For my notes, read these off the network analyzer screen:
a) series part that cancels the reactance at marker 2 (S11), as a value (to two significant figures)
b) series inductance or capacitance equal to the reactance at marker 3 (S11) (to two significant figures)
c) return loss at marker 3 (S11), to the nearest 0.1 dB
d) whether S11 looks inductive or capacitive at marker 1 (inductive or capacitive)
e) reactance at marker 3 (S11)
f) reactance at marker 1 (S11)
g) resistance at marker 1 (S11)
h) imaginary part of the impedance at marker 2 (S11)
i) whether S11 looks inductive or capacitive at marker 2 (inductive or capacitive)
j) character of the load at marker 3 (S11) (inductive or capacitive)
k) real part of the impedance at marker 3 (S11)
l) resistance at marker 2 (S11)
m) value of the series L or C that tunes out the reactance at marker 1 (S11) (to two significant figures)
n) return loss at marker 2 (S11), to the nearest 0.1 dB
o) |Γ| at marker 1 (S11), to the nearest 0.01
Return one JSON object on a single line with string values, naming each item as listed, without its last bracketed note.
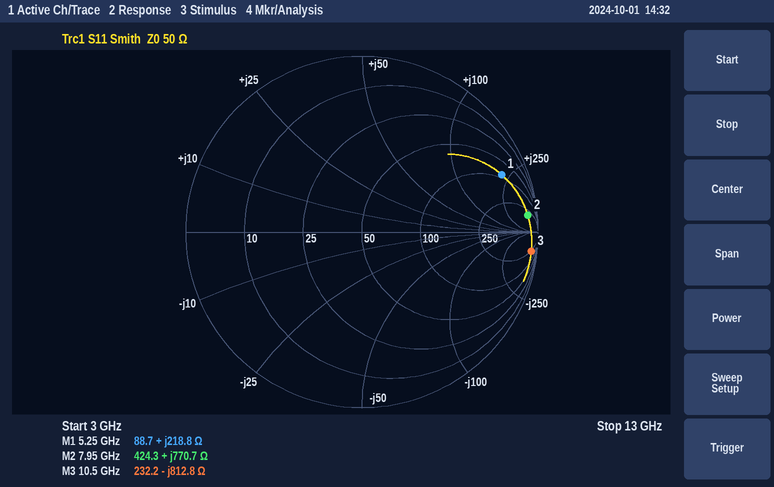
{"series part that cancels the reactance at marker 2 (S11), as a value": "26 fF", "series inductance or capacitance equal to the reactance at marker 3 (S11)": "19 fF", "return loss at marker 3 (S11), to the nearest 0.1 dB": "0.3 dB", "whether S11 looks inductive or capacitive at marker 1": "inductive", "reactance at marker 3": "-812.8 Ω", "reactance at marker 1": "+218.8 Ω", "resistance at marker 1": "88.7 Ω", "imaginary part of the impedance at marker 2": "+770.7 Ω", "whether S11 looks inductive or capacitive at marker 2": "inductive", "character of the load at marker 3 (S11)": "capacitive", "real part of the impedance at marker 3": "232.2 Ω", "resistance at marker 2": "424.3 Ω", "value of the series L or C that tunes out the reactance at marker 1 (S11)": "140 fF", "return loss at marker 2 (S11), to the nearest 0.1 dB": "0.5 dB", "|Γ| at marker 1 (S11), to the nearest 0.01": "0.86"}
